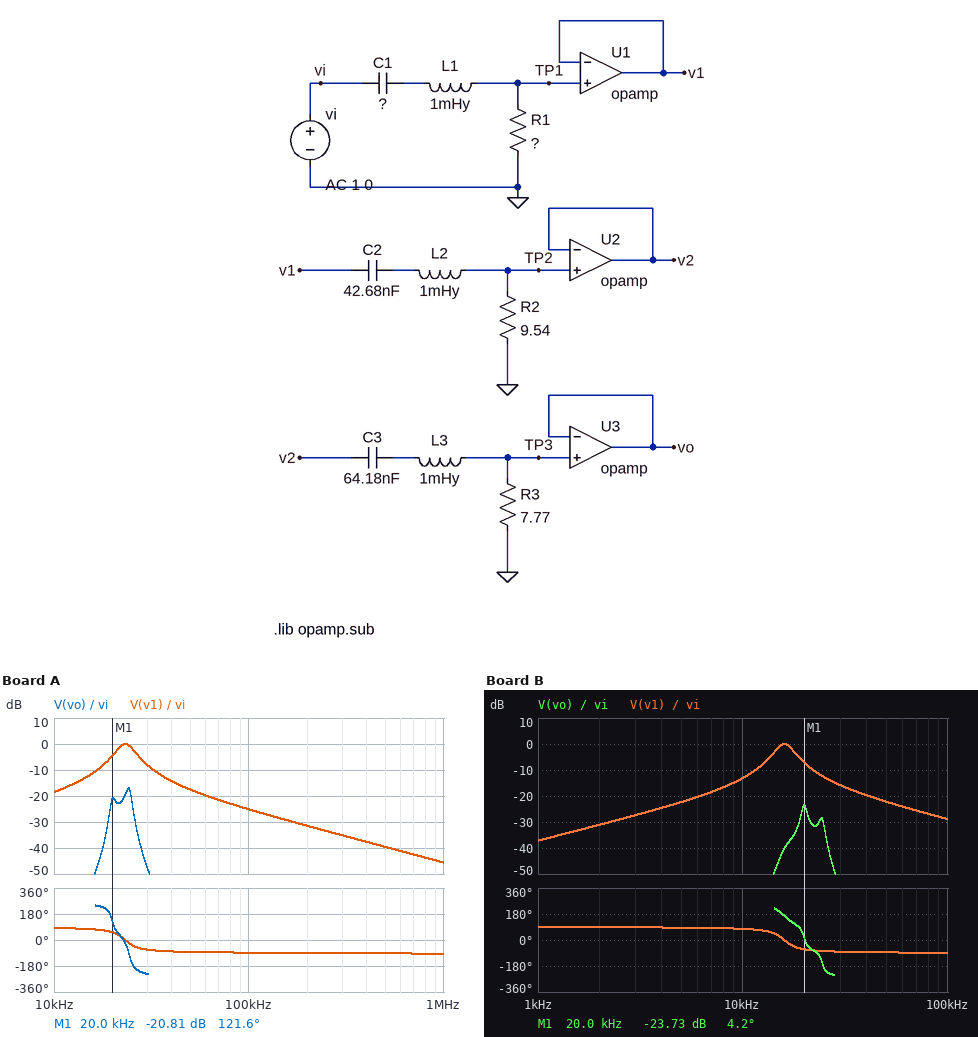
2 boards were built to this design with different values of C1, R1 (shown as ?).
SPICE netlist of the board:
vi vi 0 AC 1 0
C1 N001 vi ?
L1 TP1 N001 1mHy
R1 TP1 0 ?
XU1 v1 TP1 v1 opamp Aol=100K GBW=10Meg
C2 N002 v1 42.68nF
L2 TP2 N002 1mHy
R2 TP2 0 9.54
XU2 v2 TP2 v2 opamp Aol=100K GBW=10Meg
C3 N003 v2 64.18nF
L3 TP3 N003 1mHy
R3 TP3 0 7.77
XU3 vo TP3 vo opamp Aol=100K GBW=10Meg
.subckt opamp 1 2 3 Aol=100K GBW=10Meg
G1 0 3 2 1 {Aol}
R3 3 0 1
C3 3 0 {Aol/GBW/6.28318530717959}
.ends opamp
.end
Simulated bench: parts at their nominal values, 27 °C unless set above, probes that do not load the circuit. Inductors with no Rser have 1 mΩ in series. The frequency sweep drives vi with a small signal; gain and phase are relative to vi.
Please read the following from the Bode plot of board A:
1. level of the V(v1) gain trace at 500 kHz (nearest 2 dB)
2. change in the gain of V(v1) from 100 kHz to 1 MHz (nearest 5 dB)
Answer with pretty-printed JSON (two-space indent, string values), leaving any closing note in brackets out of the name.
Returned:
{
  "level of the V(v1) gain trace at 500 kHz": "-40 dB",
  "change in the gain of V(v1) from 100 kHz to 1 MHz": "-20 dB"
}
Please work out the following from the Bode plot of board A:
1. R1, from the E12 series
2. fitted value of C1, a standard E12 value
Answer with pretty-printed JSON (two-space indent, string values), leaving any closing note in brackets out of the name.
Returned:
{
  "R1, from the E12 series": "33 Ω",
  "fitted value of C1, a standard E12 value": "47 nF"
}
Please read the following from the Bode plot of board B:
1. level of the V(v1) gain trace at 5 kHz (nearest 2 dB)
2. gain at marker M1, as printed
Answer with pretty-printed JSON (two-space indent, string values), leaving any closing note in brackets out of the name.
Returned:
{
  "level of the V(v1) gain trace at 5 kHz": "-22 dB",
  "gain at marker M1, as printed": "-23.73 dB"
}
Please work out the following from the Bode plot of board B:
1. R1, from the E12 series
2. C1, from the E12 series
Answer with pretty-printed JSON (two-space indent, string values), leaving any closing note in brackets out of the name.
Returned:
{
  "R1, from the E12 series": "22 Ω",
  "C1, from the E12 series": "100 nF"
}
